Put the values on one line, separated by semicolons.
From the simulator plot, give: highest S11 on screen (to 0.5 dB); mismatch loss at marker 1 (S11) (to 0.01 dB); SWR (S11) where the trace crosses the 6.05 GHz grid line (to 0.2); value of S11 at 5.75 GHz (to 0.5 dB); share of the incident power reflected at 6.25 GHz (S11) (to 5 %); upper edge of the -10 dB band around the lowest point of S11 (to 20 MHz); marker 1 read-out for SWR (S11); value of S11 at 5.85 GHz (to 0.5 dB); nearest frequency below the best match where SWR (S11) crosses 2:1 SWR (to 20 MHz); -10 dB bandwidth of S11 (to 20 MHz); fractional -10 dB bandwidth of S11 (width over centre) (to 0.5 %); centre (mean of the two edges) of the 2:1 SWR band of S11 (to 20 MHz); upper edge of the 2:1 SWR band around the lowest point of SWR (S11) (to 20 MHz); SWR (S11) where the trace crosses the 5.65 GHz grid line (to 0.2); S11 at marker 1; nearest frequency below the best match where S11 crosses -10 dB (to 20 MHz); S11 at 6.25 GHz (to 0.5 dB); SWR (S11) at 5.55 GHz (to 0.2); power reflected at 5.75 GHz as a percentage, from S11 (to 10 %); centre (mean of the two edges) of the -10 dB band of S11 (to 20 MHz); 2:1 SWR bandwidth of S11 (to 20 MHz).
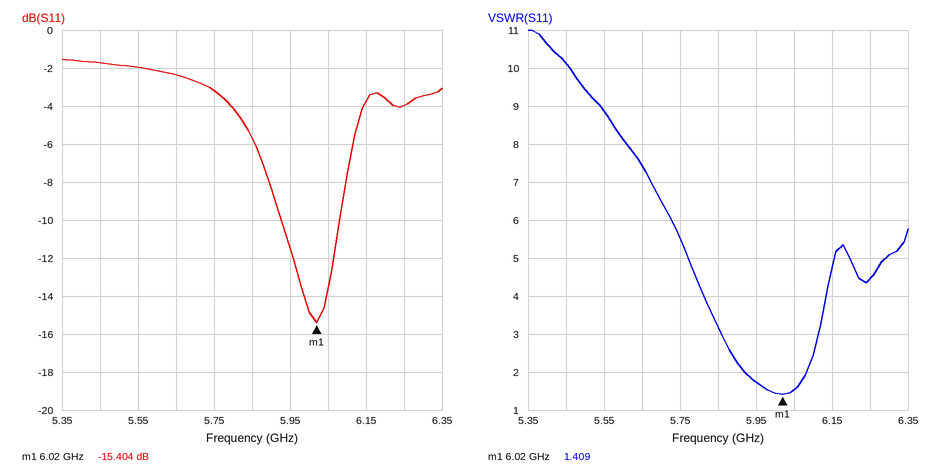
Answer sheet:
-1.5 dB; 0.13 dB; 1.6; -3.0 dB; 40 %; 6.08 GHz; 1.409; -5.5 dB; 5.92 GHz; 160 MHz; 2.5 %; 6.00 GHz; 6.08 GHz; 7.4; -15.404 dB; 5.92 GHz; -4.0 dB; 8.8; 50 %; 6.00 GHz; 160 MHz
